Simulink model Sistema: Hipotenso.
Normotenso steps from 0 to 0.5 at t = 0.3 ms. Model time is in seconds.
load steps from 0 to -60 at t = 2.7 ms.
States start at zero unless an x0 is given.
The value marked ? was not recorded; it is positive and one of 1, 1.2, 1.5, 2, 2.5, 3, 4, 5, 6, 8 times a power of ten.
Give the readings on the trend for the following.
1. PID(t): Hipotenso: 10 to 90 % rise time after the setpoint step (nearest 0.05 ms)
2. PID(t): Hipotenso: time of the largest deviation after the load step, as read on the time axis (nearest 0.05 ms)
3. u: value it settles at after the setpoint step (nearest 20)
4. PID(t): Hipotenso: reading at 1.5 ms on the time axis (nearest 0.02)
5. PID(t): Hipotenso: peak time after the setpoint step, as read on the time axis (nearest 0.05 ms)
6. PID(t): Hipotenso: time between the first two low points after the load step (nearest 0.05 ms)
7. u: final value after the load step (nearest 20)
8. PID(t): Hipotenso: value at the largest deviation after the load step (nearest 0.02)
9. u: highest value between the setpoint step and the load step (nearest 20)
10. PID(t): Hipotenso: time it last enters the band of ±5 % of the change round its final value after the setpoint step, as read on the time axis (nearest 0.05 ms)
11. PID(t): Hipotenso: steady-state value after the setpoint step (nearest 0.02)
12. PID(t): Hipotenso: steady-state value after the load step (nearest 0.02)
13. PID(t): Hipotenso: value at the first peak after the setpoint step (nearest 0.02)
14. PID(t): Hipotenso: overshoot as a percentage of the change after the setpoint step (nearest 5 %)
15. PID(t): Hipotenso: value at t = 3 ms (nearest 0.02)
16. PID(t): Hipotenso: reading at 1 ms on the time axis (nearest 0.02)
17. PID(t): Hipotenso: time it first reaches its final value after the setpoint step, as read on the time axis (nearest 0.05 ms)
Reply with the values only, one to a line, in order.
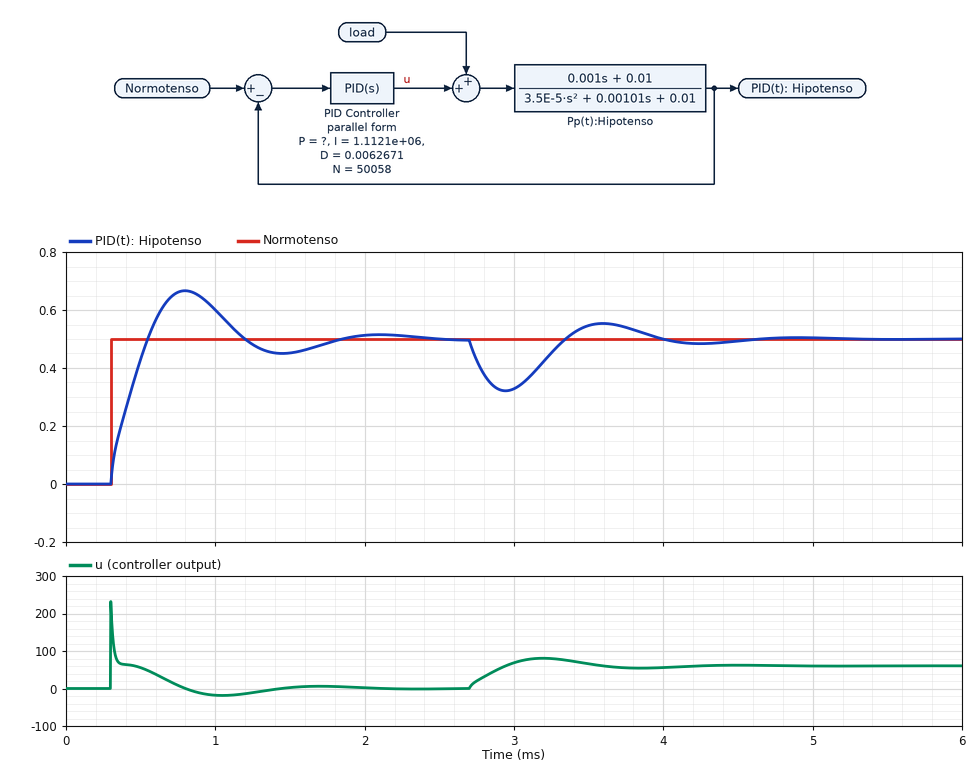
0.20 ms
2.95 ms
0
0.46
0.80 ms
1.30 ms
60
0.32
240
1.70 ms
0.50
0.50
0.66
35 %
0.32
0.60
0.55 ms
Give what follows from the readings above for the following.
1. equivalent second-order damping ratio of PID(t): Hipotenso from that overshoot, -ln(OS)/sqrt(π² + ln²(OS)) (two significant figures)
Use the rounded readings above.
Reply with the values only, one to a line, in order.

0.32
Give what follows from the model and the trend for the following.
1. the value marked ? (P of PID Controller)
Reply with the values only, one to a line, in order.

150
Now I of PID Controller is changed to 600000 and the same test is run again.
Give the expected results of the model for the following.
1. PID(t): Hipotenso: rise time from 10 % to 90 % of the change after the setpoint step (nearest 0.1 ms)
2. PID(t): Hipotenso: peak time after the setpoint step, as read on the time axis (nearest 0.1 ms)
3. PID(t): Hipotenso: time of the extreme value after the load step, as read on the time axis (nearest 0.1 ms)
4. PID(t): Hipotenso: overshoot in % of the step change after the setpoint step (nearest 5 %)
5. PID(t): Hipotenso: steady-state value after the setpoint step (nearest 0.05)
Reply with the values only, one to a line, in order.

0.3 ms
0.9 ms
3.0 ms
25 %
0.50
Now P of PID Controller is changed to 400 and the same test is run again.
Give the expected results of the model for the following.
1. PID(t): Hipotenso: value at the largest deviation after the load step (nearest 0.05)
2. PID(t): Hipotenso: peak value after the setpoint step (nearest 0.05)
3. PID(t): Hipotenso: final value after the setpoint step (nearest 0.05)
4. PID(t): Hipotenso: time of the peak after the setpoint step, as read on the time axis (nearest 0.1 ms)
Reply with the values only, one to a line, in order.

0.40
0.55
0.50
0.7 ms
